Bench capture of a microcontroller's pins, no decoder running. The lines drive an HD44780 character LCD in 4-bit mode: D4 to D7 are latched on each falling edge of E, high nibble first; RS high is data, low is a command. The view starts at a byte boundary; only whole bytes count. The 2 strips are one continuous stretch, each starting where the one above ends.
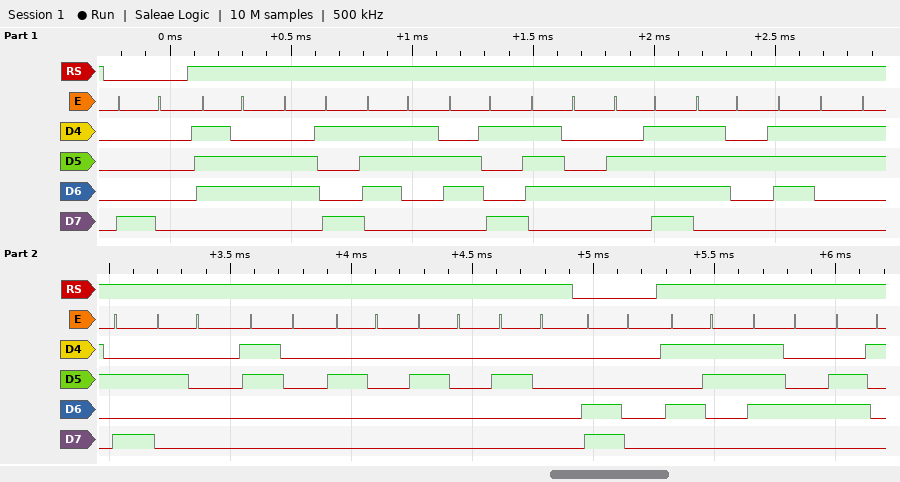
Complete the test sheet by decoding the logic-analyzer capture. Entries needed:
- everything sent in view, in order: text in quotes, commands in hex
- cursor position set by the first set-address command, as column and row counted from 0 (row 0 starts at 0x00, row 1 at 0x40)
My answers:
0x80 "visitors: 0   " 0xC0 "Sta"
column 0, row 0
